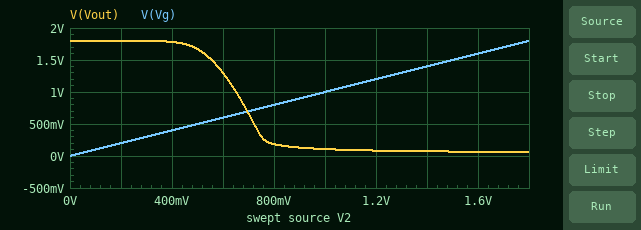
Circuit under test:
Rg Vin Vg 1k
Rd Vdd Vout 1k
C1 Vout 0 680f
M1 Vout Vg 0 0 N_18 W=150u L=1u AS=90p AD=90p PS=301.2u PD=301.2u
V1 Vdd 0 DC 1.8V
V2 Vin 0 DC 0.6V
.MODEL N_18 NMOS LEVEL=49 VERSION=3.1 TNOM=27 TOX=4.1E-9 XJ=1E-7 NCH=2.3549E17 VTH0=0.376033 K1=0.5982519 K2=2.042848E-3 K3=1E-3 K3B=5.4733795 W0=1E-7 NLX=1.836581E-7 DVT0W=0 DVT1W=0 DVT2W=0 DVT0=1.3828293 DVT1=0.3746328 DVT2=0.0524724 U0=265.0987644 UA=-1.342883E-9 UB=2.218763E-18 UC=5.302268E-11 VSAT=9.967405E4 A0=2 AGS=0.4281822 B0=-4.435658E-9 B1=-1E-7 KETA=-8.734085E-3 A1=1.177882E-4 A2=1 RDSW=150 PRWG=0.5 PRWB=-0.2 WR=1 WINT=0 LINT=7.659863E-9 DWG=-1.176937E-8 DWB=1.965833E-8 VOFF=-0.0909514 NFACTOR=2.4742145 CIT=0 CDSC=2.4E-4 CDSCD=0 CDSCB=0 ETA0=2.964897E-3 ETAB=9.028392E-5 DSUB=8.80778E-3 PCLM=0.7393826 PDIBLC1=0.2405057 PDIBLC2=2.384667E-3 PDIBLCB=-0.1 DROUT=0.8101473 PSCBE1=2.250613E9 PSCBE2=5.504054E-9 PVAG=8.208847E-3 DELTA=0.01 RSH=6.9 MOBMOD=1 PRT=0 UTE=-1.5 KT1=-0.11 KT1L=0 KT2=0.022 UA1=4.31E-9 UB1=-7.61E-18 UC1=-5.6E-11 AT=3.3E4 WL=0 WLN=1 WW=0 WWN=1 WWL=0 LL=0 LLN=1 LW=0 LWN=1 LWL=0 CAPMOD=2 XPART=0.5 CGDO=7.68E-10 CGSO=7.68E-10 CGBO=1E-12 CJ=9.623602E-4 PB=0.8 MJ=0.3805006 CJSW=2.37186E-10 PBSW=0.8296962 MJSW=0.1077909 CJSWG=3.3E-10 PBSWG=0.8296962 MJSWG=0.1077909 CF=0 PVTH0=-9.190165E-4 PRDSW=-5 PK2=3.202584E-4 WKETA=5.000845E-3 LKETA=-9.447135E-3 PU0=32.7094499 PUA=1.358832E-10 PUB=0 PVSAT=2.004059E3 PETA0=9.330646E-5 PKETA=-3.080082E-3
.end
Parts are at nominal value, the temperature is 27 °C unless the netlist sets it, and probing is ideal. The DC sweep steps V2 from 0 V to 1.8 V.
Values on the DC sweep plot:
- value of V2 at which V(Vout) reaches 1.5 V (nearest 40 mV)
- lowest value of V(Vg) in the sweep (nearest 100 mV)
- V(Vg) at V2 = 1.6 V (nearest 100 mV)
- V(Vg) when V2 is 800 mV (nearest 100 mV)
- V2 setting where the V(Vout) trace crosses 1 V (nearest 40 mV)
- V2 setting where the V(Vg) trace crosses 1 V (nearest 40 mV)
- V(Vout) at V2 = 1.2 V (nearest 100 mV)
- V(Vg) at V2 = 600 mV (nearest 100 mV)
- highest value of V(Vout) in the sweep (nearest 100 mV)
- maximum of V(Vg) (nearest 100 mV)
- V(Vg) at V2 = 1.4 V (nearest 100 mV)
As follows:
560 mV
0 V
1.6 V
800 mV
640 mV
1.00 V
100 mV
600 mV
1.8 V
1.8 V
1.4 V
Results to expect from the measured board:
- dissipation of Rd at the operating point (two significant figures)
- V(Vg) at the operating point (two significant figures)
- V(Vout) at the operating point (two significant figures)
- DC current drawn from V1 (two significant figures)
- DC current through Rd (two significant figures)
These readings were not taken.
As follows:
250 µW
600 mV
1.3 V
500 µA
500 µA
